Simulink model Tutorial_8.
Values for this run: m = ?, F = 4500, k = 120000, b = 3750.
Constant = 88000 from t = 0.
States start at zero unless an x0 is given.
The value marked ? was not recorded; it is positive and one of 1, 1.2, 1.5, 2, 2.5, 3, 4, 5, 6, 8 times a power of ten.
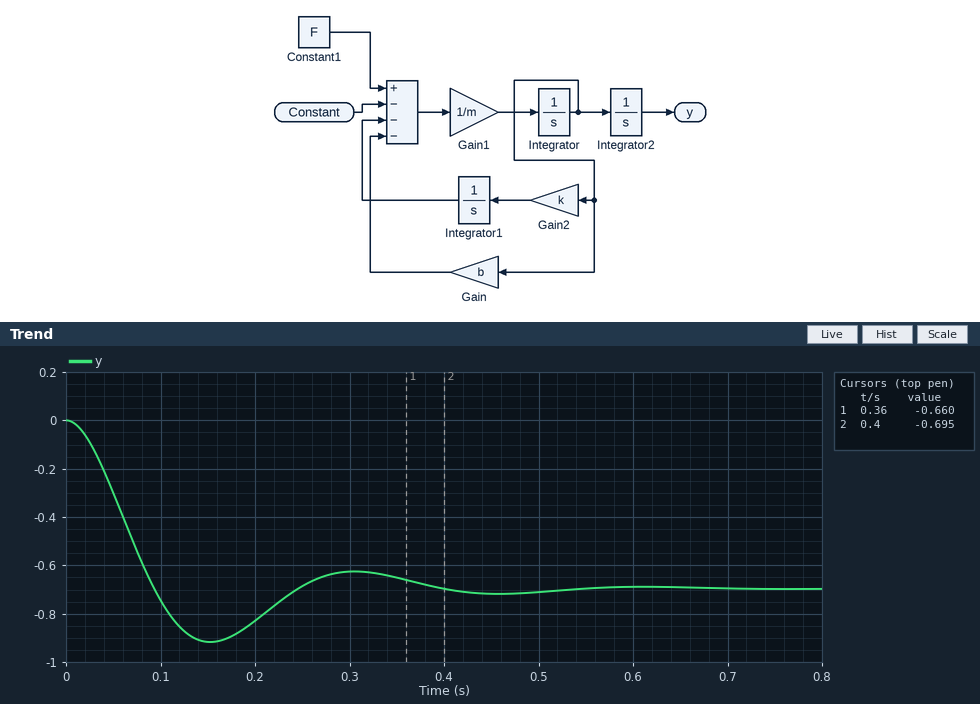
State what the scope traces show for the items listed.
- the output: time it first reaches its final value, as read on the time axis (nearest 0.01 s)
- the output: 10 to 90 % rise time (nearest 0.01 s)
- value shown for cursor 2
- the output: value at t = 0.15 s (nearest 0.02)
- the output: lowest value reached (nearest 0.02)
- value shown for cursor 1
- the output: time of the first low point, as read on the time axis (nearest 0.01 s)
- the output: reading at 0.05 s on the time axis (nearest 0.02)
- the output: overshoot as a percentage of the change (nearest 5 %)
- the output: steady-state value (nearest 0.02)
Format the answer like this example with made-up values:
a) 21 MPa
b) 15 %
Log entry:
a) 0.09 s
b) 0.06 s
c) -0.695
d) -0.92
e) -0.92
f) -0.660
g) 0.15 s
h) -0.30
i) 30 %
j) -0.70
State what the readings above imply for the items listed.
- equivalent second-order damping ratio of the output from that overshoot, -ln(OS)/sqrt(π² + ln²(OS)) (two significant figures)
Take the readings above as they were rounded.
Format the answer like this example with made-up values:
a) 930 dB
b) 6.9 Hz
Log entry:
a) 0.36
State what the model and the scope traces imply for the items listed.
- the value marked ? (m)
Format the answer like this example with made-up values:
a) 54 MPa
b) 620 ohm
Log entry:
a) 250
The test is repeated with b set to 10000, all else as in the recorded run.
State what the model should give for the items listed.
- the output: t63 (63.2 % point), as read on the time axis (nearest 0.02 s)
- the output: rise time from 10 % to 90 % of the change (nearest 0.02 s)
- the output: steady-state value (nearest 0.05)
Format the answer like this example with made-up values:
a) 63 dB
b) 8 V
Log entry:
a) 0.10 s
b) 0.14 s
c) -0.70
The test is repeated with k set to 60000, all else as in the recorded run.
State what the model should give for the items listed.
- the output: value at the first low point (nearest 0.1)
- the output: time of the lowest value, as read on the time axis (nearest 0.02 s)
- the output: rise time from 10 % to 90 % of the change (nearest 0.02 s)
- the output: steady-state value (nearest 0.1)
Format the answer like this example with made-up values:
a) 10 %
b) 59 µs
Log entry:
a) -1.6
b) 0.24 s
c) 0.10 s
d) -1.4
